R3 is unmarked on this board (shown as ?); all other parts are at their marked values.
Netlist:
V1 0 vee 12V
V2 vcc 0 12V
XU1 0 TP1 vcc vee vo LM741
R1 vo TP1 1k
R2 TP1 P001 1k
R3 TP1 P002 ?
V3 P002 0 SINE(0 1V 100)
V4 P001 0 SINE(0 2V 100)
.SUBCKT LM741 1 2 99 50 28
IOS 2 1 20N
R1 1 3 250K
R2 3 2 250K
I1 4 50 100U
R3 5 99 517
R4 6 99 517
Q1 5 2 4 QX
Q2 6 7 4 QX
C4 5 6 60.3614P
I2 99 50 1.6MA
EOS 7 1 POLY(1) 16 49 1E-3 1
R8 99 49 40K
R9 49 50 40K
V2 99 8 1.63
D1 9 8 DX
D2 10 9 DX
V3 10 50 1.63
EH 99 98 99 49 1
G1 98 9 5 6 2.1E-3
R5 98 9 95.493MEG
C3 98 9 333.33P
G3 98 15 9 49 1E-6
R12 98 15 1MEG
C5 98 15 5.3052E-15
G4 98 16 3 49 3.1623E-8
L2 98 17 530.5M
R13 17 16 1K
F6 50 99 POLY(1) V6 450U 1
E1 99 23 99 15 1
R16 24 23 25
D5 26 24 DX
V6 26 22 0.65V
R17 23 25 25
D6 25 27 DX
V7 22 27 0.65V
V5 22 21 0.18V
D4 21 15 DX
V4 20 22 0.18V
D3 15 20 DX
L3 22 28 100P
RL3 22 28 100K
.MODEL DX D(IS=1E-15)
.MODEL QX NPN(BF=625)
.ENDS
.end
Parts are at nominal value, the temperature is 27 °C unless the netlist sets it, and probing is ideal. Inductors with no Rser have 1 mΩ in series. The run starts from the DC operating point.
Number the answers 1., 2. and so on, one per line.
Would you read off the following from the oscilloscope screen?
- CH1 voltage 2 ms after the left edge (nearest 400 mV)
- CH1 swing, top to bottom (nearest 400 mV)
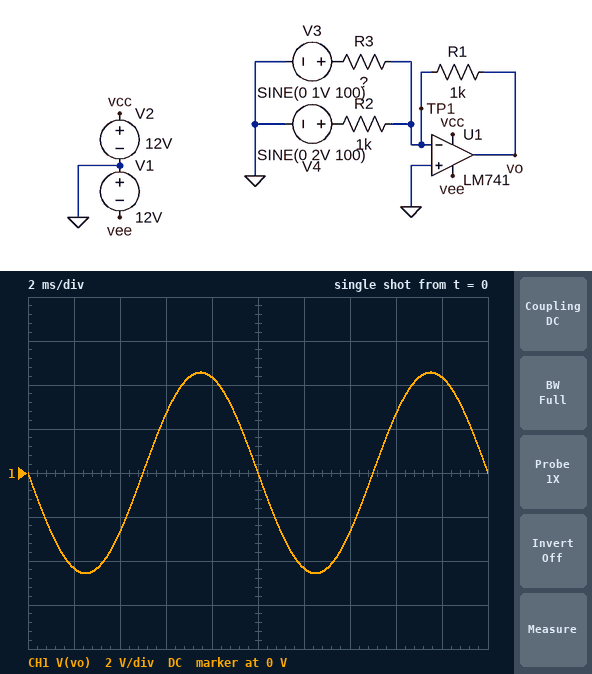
1. -4.4 V
2. 9.2 V
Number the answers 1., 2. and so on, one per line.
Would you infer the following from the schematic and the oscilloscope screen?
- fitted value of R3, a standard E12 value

1. 390 Ω
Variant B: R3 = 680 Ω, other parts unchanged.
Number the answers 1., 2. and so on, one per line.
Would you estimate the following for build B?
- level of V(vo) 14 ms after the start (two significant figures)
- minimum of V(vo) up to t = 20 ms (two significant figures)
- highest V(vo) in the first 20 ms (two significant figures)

1. -2.0 V
2. -3.5 V
3. 3.5 V
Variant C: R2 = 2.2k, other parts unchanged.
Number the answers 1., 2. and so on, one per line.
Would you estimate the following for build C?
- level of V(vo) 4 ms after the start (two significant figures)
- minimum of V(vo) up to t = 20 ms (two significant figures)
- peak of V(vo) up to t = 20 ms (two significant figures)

1. -2.0 V
2. -3.5 V
3. 3.5 V
